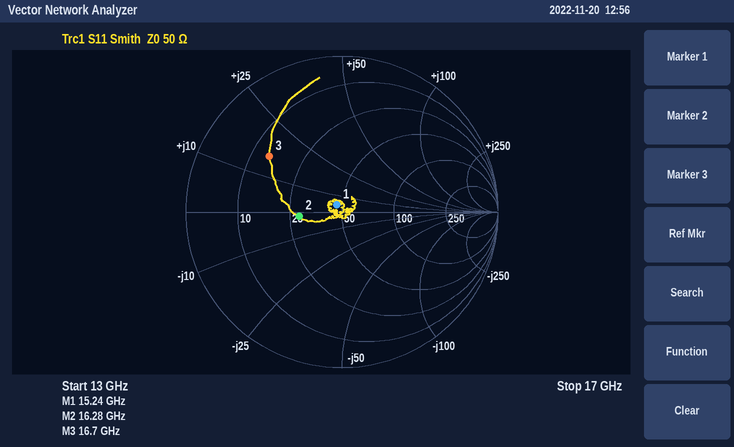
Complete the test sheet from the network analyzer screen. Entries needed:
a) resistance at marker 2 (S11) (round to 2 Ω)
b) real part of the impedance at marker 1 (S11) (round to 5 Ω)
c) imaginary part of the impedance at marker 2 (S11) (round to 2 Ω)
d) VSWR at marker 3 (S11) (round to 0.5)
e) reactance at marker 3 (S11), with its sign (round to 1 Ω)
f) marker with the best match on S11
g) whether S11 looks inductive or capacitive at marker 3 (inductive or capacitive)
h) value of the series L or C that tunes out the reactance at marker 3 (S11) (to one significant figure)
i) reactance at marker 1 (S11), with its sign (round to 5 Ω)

28 Ω
45 Ω
-2 Ω
4.0
+16 Ω
marker 1
inductive
600 fF
+5 Ω
